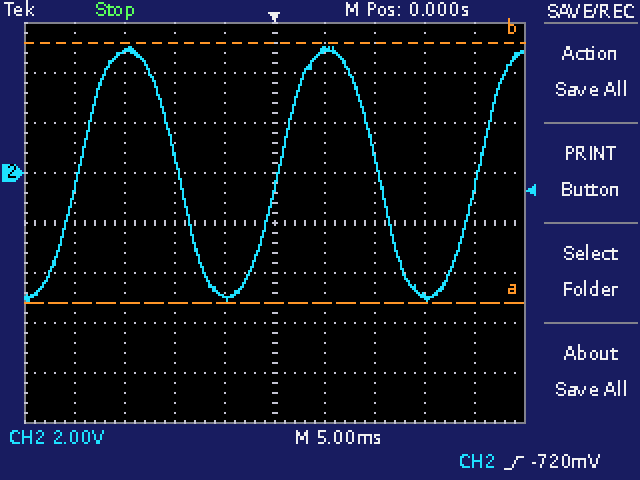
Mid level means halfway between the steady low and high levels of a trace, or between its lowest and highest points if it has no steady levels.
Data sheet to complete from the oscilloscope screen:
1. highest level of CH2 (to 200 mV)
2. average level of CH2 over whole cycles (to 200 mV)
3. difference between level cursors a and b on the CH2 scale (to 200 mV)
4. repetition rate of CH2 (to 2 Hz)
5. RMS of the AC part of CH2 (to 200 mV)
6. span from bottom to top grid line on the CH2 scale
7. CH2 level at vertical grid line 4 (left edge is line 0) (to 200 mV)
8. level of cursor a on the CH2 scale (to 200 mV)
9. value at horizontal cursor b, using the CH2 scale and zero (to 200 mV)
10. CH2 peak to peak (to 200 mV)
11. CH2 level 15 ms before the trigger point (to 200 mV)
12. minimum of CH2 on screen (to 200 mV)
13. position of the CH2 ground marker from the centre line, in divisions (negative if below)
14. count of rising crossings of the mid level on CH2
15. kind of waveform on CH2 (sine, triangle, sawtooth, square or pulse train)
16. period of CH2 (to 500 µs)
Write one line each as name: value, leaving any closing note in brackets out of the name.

highest level of CH2: 5.0 V
average level of CH2 over whole cycles: 0.0 V
difference between level cursors a and b on the CH2 scale: 10.4 V
repetition rate of CH2: 50 Hz
RMS of the AC part of CH2: 3.6 V
span from bottom to top grid line on the CH2 scale: 16 V
CH2 level at vertical grid line 4 (left edge is line 0): -5.0 V
level of cursor a on the CH2 scale: -5.2 V
value at horizontal cursor b, using the CH2 scale and zero: 5.2 V
CH2 peak to peak: 10.2 V
CH2 level 15 ms before the trigger point: 4.8 V
minimum of CH2 on screen: -5.2 V
position of the CH2 ground marker from the centre line, in divisions: +1.0 div
count of rising crossings of the mid level on CH2: 3
kind of waveform on CH2: sine
period of CH2: 20.0 ms
